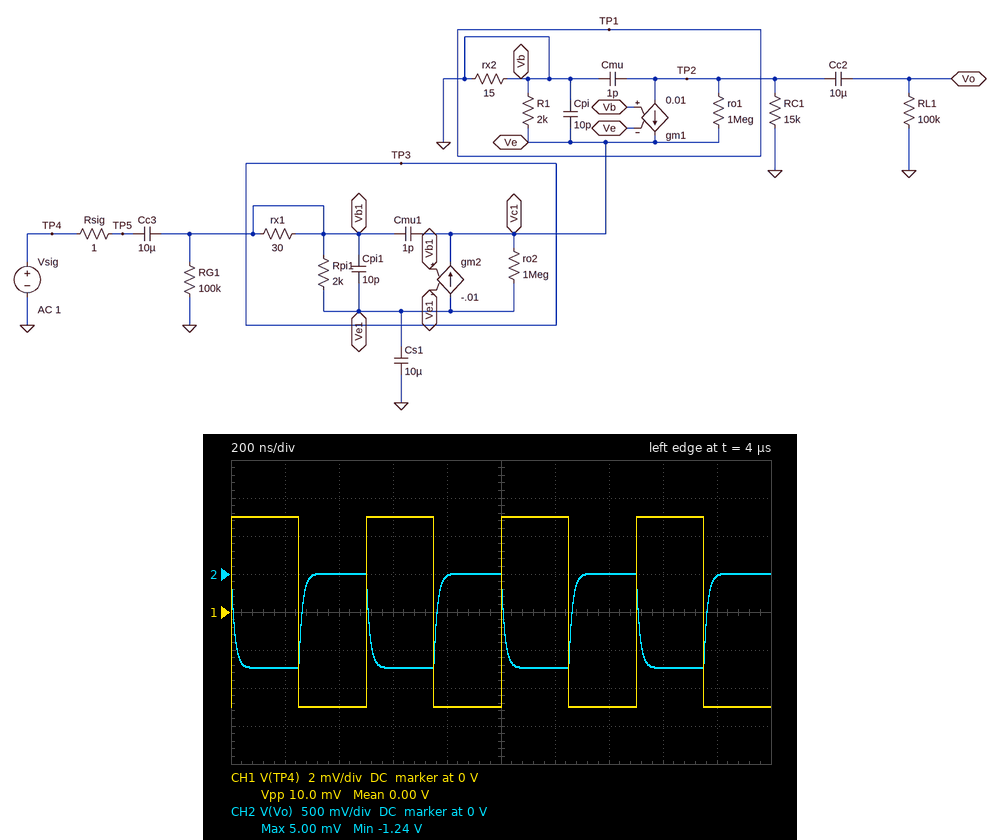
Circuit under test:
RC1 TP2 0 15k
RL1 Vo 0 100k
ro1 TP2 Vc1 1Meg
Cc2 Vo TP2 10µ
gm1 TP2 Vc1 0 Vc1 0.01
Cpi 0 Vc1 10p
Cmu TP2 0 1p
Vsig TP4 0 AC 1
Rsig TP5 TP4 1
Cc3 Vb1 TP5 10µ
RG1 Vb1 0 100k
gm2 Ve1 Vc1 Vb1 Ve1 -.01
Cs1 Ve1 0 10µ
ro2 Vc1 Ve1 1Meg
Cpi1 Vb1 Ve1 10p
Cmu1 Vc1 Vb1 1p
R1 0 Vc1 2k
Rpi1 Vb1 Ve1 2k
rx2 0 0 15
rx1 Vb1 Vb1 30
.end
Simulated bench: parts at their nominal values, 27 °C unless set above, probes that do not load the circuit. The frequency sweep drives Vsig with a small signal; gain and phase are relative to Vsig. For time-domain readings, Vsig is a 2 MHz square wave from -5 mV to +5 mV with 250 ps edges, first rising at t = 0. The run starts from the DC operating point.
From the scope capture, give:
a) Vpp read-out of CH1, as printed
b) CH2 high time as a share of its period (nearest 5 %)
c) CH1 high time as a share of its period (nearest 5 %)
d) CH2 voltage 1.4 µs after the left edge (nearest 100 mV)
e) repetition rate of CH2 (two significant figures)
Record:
10.0 mV
50 %
50 %
0 V
2.0 MHz
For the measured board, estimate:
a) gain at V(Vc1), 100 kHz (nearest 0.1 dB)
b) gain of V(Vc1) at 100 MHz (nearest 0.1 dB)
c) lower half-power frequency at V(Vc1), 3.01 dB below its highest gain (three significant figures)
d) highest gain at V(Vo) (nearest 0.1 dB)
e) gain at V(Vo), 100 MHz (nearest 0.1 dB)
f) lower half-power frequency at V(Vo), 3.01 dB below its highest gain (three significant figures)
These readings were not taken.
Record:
-0.3 dB
-2.0 dB
175 Hz
41.9 dB
22.0 dB
175 Hz
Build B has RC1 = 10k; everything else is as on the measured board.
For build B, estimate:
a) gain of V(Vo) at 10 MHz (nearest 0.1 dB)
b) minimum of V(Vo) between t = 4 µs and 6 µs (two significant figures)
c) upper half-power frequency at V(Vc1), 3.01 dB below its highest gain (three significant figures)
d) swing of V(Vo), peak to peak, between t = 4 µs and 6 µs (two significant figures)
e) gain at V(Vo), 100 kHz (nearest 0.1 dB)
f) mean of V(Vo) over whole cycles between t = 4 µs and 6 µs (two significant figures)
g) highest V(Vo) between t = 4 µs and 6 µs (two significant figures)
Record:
37.5 dB
-860 mV
150 MHz
870 mV
38.7 dB
-430 mV
3.0 mV
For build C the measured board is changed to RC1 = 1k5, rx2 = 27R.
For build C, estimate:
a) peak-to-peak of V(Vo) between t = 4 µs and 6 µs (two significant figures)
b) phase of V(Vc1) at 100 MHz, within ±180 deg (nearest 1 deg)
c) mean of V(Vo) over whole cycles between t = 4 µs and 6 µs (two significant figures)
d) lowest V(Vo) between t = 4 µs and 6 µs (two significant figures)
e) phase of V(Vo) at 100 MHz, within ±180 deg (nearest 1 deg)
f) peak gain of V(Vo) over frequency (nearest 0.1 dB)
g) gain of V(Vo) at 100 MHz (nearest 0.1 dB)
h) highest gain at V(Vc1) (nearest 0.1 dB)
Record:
140 mV
143 deg
-70 mV
-140 mV
100 deg
23.0 dB
18.7 dB
-0.4 dB
